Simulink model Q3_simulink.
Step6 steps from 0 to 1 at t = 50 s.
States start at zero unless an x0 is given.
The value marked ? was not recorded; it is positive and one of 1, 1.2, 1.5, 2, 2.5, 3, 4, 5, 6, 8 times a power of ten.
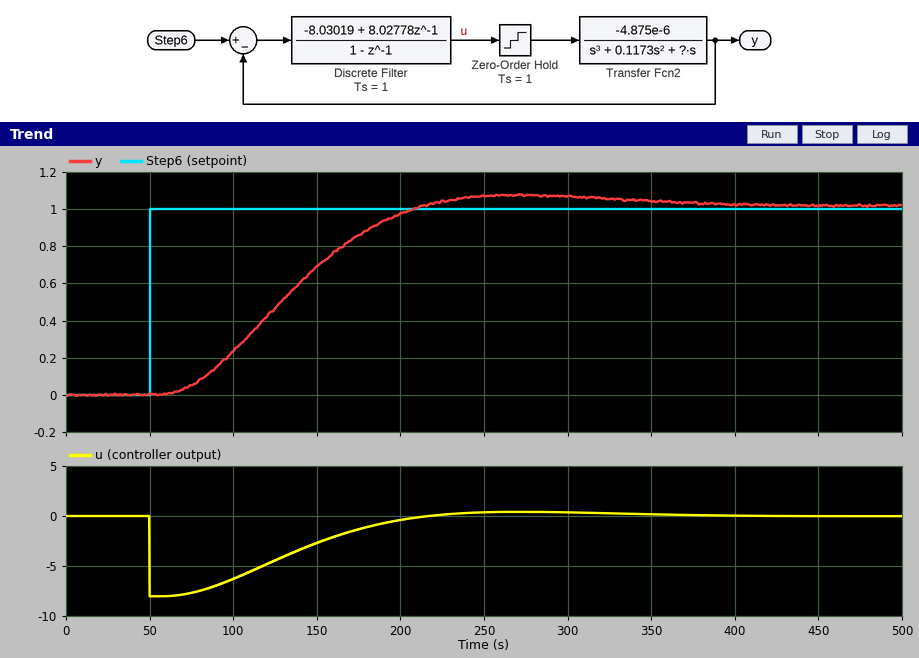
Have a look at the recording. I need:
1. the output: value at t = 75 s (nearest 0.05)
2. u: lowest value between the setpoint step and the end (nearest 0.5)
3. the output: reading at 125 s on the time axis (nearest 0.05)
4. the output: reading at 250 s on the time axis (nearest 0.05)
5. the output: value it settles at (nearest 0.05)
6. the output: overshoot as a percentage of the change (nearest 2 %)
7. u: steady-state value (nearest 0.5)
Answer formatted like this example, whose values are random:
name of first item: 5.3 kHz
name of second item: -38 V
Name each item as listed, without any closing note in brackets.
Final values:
the output: value at t = 75 s: 0.05
u: lowest value between the setpoint step and the end: -8.0
the output: reading at 125 s on the time axis: 0.45
the output: reading at 250 s on the time axis: 1.05
the output: value it settles at: 1.00
the output: overshoot as a percentage of the change: 6 %
u: steady-state value: 0.0
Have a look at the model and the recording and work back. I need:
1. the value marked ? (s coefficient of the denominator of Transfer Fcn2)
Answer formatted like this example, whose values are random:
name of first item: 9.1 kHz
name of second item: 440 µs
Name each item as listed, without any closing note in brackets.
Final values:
the value marked ?: 0.003
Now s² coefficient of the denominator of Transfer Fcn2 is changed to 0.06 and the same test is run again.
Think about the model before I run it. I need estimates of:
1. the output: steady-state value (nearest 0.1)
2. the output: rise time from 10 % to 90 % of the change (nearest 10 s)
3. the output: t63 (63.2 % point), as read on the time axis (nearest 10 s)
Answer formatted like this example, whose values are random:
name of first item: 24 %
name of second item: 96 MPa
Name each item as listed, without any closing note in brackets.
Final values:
the output: steady-state value: 1.0
the output: rise time from 10 % to 90 % of the change: 100 s
the output: t63 (63.2 % point), as read on the time axis: 130 s
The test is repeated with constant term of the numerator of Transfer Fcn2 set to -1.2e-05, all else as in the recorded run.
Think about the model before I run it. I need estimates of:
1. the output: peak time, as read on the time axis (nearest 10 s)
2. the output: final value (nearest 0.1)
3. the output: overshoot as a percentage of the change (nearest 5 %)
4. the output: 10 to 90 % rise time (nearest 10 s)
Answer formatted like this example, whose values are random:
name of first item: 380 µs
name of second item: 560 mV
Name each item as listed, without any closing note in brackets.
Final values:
the output: peak time, as read on the time axis: 170 s
the output: final value: 1.0
the output: overshoot as a percentage of the change: 35 %
the output: 10 to 90 % rise time: 50 s
